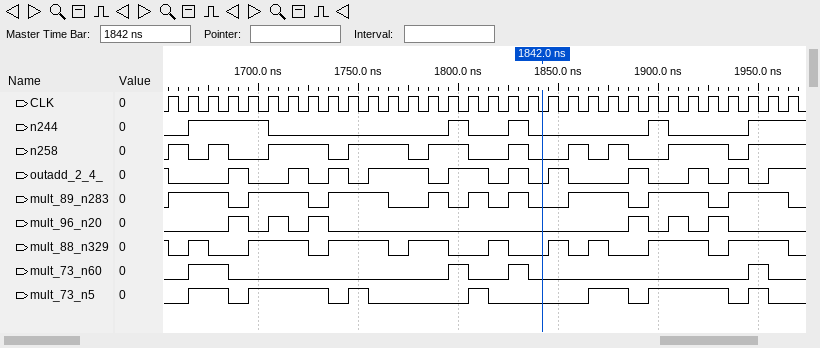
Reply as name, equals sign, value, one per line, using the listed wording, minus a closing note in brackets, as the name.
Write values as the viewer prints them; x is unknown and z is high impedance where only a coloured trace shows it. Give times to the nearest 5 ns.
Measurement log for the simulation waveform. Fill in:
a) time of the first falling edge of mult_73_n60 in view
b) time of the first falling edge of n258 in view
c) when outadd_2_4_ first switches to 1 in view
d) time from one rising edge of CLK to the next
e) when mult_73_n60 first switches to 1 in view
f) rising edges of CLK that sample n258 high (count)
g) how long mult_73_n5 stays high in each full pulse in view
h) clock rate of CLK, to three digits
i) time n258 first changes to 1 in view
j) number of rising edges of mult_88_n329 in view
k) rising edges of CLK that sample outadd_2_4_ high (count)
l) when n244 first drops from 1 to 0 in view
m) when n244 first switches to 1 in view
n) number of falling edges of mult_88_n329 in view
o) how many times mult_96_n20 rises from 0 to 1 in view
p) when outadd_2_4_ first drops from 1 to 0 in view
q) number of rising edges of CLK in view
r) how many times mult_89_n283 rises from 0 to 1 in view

time of the first falling edge of mult_73_n60 in view = 1685 ns
time of the first falling edge of n258 in view = 1665 ns
when outadd_2_4_ first switches to 1 in view = 1685 ns
time from one rising edge of CLK to the next = 10 ns
when mult_73_n60 first switches to 1 in view = 1665 ns
rising edges of CLK that sample n258 high = 18
how long mult_73_n5 stays high in each full pulse in view = 20 ns, 40 ns, 10 ns, 10 ns, 20 ns, 40 ns, 10 ns
clock rate of CLK, to three digits = 100 MHz
time n258 first changes to 1 in view = 1655 ns
number of rising edges of mult_88_n329 in view = 9
rising edges of CLK that sample outadd_2_4_ high = 15
when n244 first drops from 1 to 0 in view = 1705 ns
when n244 first switches to 1 in view = 1665 ns
number of falling edges of mult_88_n329 in view = 10
how many times mult_96_n20 rises from 0 to 1 in view = 6
when outadd_2_4_ first drops from 1 to 0 in view = 1655 ns
number of rising edges of CLK in view = 32
how many times mult_89_n283 rises from 0 to 1 in view = 9
